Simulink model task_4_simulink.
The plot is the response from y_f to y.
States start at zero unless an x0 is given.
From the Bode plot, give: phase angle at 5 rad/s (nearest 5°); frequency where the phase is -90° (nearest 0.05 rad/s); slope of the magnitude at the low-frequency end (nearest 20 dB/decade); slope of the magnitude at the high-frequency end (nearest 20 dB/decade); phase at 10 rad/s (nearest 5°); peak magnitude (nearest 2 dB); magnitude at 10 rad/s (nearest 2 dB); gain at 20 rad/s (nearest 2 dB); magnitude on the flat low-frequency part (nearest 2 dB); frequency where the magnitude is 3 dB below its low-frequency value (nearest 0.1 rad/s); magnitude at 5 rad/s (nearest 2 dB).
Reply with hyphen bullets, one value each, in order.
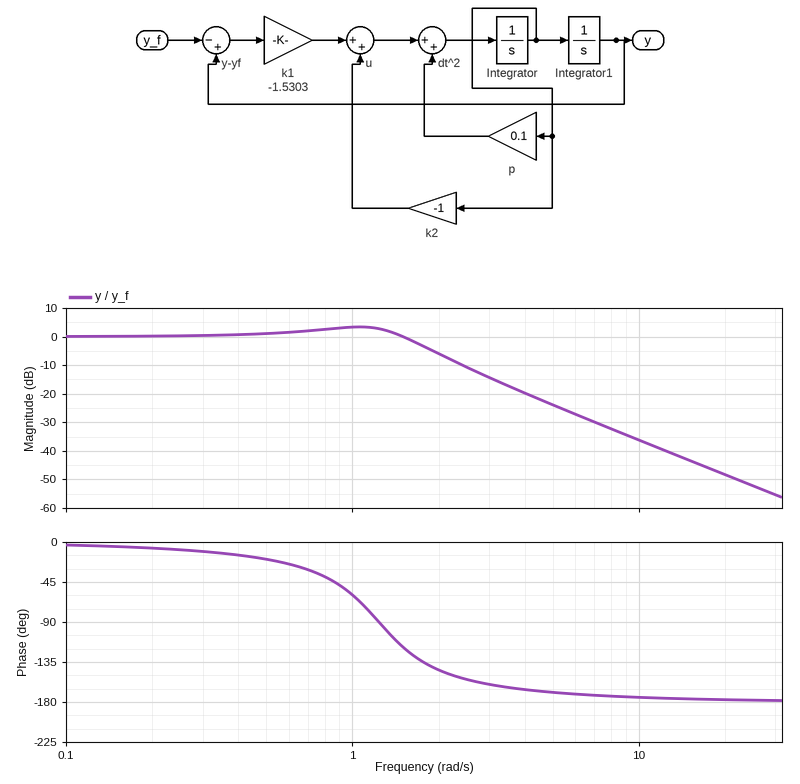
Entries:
- -170°
- 1.25 rad/s
- 0 dB/decade
- -40 dB/decade
- -175°
- 4 dB
- -36 dB
- -48 dB
- 0 dB
- 1.7 rad/s
- -24 dB
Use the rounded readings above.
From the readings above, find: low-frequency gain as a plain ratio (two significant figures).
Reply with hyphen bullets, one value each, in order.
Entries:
- 1.0
